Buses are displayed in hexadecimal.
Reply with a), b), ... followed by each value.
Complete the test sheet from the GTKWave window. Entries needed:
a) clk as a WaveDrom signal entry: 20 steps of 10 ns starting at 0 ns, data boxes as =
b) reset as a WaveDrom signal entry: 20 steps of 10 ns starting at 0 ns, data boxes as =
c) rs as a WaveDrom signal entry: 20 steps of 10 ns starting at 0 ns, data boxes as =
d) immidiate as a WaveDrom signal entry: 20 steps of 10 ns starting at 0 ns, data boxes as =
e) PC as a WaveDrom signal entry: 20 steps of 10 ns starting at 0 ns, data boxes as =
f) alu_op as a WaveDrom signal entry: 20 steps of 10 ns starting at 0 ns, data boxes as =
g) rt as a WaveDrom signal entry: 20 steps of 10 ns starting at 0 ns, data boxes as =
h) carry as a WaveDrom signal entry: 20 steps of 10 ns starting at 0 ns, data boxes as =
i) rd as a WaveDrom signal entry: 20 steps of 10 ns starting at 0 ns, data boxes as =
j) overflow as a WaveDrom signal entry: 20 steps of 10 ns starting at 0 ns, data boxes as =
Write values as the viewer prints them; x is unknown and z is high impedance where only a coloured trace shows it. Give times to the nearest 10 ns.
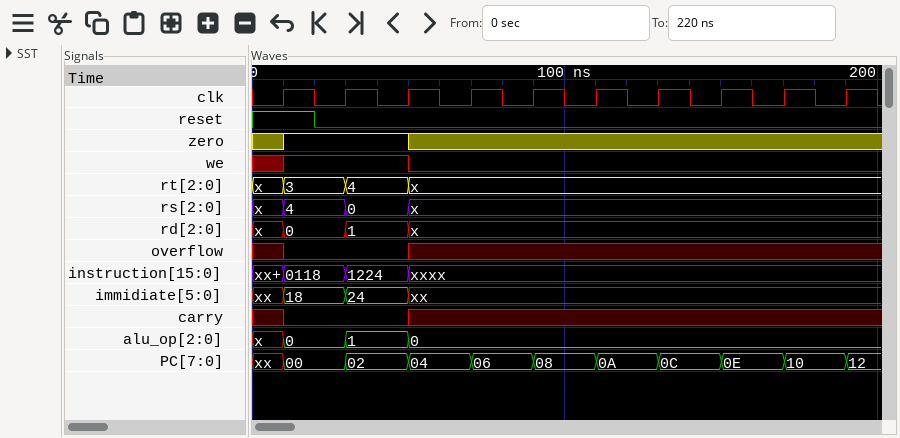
a) {name: 'clk', wave: '01010101010101010101'}
b) {name: 'reset', wave: '1.0.................'}
c) {name: 'rs', wave: 'x=.=.x..............', data: '4 0'}
d) {name: 'immidiate', wave: 'x=.=.x..............', data: '18 24'}
e) {name: 'PC', wave: 'x=.=.=.=.=.=.=.=.=.=', data: '00 02 04 06 08 0A 0C 0E 10 12'}
f) {name: 'alu_op', wave: 'x=.=.=..............', data: '0 1 0'}
g) {name: 'rt', wave: 'x=.=.x..............', data: '3 4'}
h) {name: 'carry', wave: 'x0...x..............'}
i) {name: 'rd', wave: 'x=.=.x..............', data: '0 1'}
j) {name: 'overflow', wave: 'x0...x..............'}
